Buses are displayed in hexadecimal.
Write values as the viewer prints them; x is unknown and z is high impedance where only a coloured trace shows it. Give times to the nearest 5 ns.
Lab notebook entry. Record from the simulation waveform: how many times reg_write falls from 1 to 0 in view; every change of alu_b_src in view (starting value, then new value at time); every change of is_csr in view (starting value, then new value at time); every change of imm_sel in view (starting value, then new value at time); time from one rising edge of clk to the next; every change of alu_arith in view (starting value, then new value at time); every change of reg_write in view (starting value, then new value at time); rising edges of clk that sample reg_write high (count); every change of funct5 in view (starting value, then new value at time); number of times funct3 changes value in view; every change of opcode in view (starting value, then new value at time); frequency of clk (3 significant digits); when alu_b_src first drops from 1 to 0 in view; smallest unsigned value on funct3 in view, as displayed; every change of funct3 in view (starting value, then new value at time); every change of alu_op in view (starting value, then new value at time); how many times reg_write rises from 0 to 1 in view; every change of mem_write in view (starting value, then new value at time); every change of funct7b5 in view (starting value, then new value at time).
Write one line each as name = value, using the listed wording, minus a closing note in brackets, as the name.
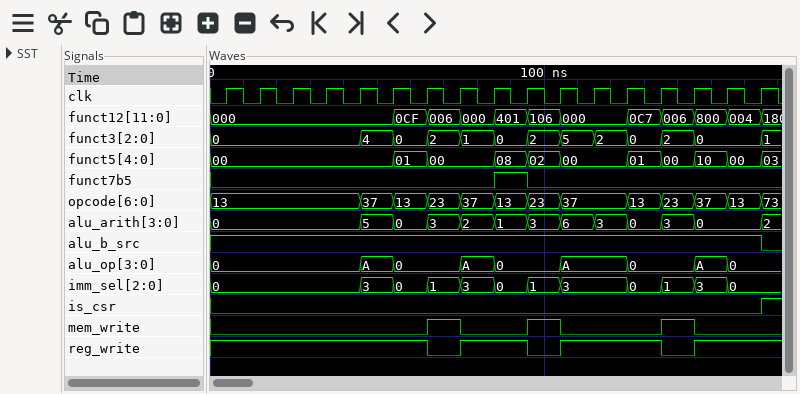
how many times reg_write falls from 1 to 0 in view = 3
every change of alu_b_src in view = 1, 0 at 165 ns
every change of is_csr in view = 0, 1 at 165 ns
every change of imm_sel in view = 0, 3 at 45 ns, 0 at 55 ns, 1 at 65 ns, 3 at 75 ns, 0 at 85 ns, 1 at 95 ns, 3 at 105 ns, 0 at 125 ns, 1 at 135 ns, 3 at 145 ns, 0 at 155 ns
time from one rising edge of clk to the next = 10 ns
every change of alu_arith in view = 0, 5 at 45 ns, 0 at 55 ns, 3 at 65 ns, 2 at 75 ns, 1 at 85 ns, 3 at 95 ns, 6 at 105 ns, 3 at 115 ns, 0 at 125 ns, 3 at 135 ns, 0 at 145 ns, 2 at 165 ns
every change of reg_write in view = 1, 0 at 65 ns, 1 at 75 ns, 0 at 95 ns, 1 at 105 ns, 0 at 135 ns, 1 at 145 ns
rising edges of clk that sample reg_write high = 14
every change of funct5 in view = 00, 01 at 55 ns, 00 at 65 ns, 08 at 85 ns, 02 at 95 ns, 00 at 105 ns, 01 at 125 ns, 00 at 135 ns, 10 at 145 ns, 00 at 155 ns, 03 at 165 ns
number of times funct3 changes value in view = 12
every change of opcode in view = 13, 37 at 45 ns, 13 at 55 ns, 23 at 65 ns, 37 at 75 ns, 13 at 85 ns, 23 at 95 ns, 37 at 105 ns, 13 at 125 ns, 23 at 135 ns, 37 at 145 ns, 13 at 155 ns, 73 at 165 ns
frequency of clk = 100 MHz
when alu_b_src first drops from 1 to 0 in view = 165 ns
smallest unsigned value on funct3 in view, as displayed = 0
every change of funct3 in view = 0, 4 at 45 ns, 0 at 55 ns, 2 at 65 ns, 1 at 75 ns, 0 at 85 ns, 2 at 95 ns, 5 at 105 ns, 2 at 115 ns, 0 at 125 ns, 2 at 135 ns, 0 at 145 ns, 1 at 165 ns
every change of alu_op in view = 0, A at 45 ns, 0 at 55 ns, A at 75 ns, 0 at 85 ns, A at 105 ns, 0 at 125 ns, A at 145 ns, 0 at 155 ns
how many times reg_write rises from 0 to 1 in view = 3
every change of mem_write in view = 0, 1 at 65 ns, 0 at 75 ns, 1 at 95 ns, 0 at 105 ns, 1 at 135 ns, 0 at 145 ns
every change of funct7b5 in view = 0, 1 at 85 ns, 0 at 95 ns
